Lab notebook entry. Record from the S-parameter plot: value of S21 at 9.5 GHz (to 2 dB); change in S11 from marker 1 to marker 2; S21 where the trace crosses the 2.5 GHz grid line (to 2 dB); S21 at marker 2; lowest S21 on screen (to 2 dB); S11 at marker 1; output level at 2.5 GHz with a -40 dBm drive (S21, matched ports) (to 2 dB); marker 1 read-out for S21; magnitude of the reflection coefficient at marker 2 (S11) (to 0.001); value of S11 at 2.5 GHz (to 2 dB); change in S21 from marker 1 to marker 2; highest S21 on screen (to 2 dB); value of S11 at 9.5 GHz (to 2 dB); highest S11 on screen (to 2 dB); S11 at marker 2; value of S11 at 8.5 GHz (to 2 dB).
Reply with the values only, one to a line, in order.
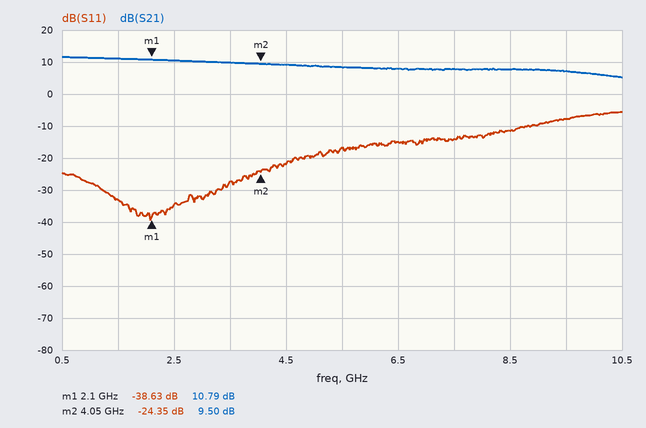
8 dB
14.28 dB
10 dB
9.50 dB
6 dB
-38.63 dB
-30 dBm
10.79 dB
0.061
-34 dB
-1.29 dB
12 dB
-8 dB
-6 dB
-24.35 dB
-12 dB
